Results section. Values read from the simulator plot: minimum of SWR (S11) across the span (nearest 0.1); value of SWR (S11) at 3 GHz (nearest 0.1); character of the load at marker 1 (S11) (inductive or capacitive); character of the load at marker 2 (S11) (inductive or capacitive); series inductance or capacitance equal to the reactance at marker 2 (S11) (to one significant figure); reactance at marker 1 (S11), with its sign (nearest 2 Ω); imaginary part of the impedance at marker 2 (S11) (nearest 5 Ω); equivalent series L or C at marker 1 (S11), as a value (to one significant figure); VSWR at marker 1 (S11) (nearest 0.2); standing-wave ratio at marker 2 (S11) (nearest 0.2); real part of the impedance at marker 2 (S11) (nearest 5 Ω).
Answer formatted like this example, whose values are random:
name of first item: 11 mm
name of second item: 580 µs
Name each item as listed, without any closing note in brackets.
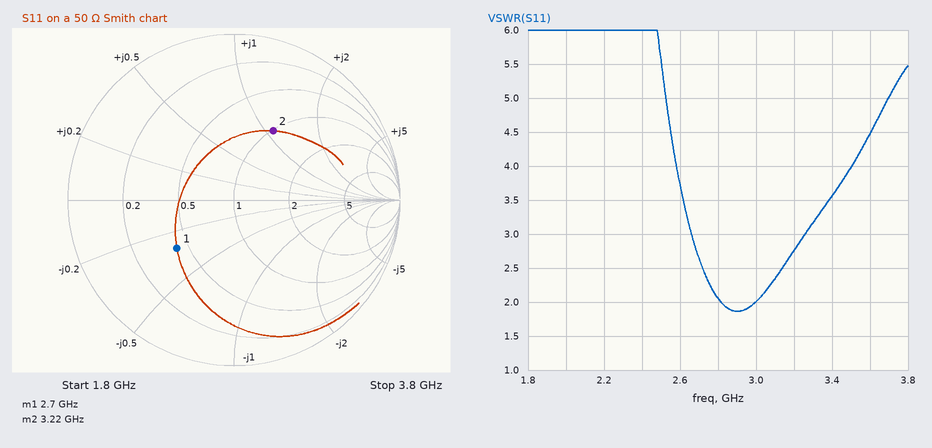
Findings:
minimum of SWR (S11) across the span: 1.9
value of SWR (S11) at 3 GHz: 2.0
character of the load at marker 1 (S11): capacitive
character of the load at marker 2 (S11): inductive
series inductance or capacitance equal to the reactance at marker 2 (S11): 3 nH
reactance at marker 1 (S11), with its sign: -16 Ω
imaginary part of the impedance at marker 2 (S11): +55 Ω
equivalent series L or C at marker 1 (S11), as a value: 4 pF
VSWR at marker 1 (S11): 2.6
standing-wave ratio at marker 2 (S11): 2.8
real part of the impedance at marker 2 (S11): 50 Ω
